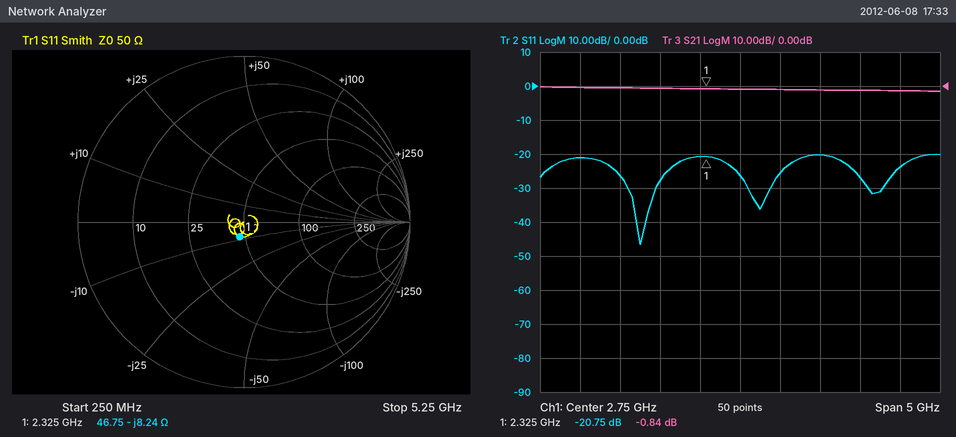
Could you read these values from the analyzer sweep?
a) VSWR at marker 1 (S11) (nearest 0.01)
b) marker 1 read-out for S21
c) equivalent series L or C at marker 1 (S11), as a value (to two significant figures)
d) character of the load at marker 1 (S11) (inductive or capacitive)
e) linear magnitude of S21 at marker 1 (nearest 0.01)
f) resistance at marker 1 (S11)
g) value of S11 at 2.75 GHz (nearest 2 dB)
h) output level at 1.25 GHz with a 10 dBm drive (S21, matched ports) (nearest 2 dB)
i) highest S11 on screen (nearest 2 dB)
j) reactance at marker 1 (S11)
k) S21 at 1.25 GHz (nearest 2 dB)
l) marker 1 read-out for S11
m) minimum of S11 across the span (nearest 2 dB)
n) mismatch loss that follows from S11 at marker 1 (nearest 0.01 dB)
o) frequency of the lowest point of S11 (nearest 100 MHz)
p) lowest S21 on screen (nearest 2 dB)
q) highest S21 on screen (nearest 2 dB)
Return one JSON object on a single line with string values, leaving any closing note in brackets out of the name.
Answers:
{"VSWR at marker 1 (S11)": "1.20", "marker 1 read-out for S21": "-0.84 dB", "equivalent series L or C at marker 1 (S11), as a value": "8.3 pF", "character of the load at marker 1 (S11)": "capacitive", "linear magnitude of S21 at marker 1": "0.91", "resistance at marker 1": "46.75 Ω", "value of S11 at 2.75 GHz": "-26 dB", "output level at 1.25 GHz with a 10 dBm drive (S21, matched ports)": "10 dBm", "highest S11 on screen": "-20 dB", "reactance at marker 1": "-8.24 Ω", "S21 at 1.25 GHz": "0 dB", "marker 1 read-out for S11": "-20.75 dB", "minimum of S11 across the span": "-46 dB", "mismatch loss that follows from S11 at marker 1": "0.04 dB", "frequency of the lowest point of S11": "1.5 GHz", "lowest S21 on screen": "-2 dB", "highest S21 on screen": "0 dB"}
